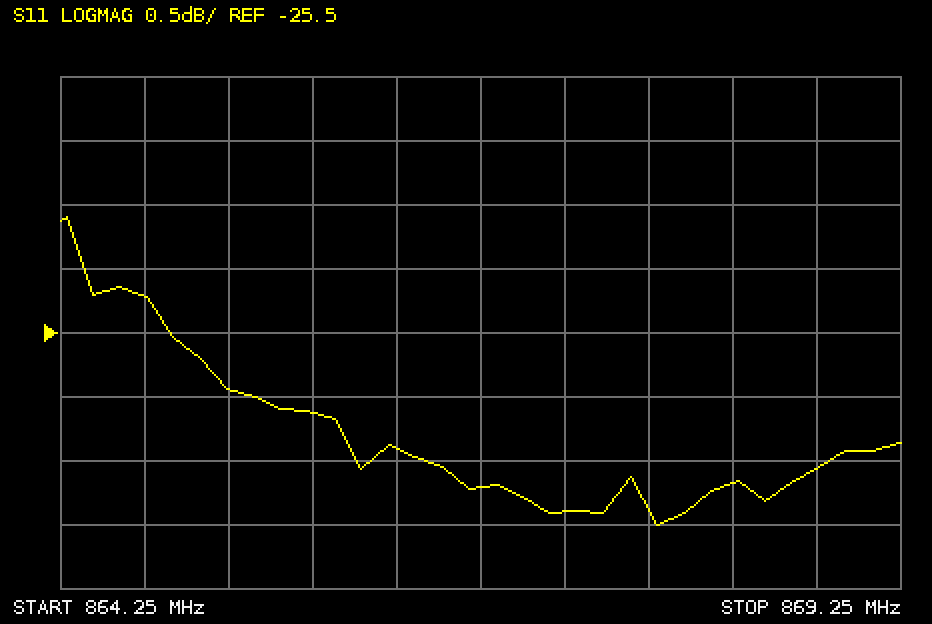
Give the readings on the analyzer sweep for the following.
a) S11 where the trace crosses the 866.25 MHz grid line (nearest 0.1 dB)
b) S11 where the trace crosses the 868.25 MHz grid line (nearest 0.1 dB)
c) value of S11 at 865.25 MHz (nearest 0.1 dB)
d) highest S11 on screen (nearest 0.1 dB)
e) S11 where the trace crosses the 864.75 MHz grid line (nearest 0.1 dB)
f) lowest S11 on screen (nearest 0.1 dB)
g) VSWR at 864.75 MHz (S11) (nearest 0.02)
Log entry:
-26.4 dB
-26.7 dB
-25.9 dB
-24.6 dB
-25.2 dB
-27.0 dB
1.12
